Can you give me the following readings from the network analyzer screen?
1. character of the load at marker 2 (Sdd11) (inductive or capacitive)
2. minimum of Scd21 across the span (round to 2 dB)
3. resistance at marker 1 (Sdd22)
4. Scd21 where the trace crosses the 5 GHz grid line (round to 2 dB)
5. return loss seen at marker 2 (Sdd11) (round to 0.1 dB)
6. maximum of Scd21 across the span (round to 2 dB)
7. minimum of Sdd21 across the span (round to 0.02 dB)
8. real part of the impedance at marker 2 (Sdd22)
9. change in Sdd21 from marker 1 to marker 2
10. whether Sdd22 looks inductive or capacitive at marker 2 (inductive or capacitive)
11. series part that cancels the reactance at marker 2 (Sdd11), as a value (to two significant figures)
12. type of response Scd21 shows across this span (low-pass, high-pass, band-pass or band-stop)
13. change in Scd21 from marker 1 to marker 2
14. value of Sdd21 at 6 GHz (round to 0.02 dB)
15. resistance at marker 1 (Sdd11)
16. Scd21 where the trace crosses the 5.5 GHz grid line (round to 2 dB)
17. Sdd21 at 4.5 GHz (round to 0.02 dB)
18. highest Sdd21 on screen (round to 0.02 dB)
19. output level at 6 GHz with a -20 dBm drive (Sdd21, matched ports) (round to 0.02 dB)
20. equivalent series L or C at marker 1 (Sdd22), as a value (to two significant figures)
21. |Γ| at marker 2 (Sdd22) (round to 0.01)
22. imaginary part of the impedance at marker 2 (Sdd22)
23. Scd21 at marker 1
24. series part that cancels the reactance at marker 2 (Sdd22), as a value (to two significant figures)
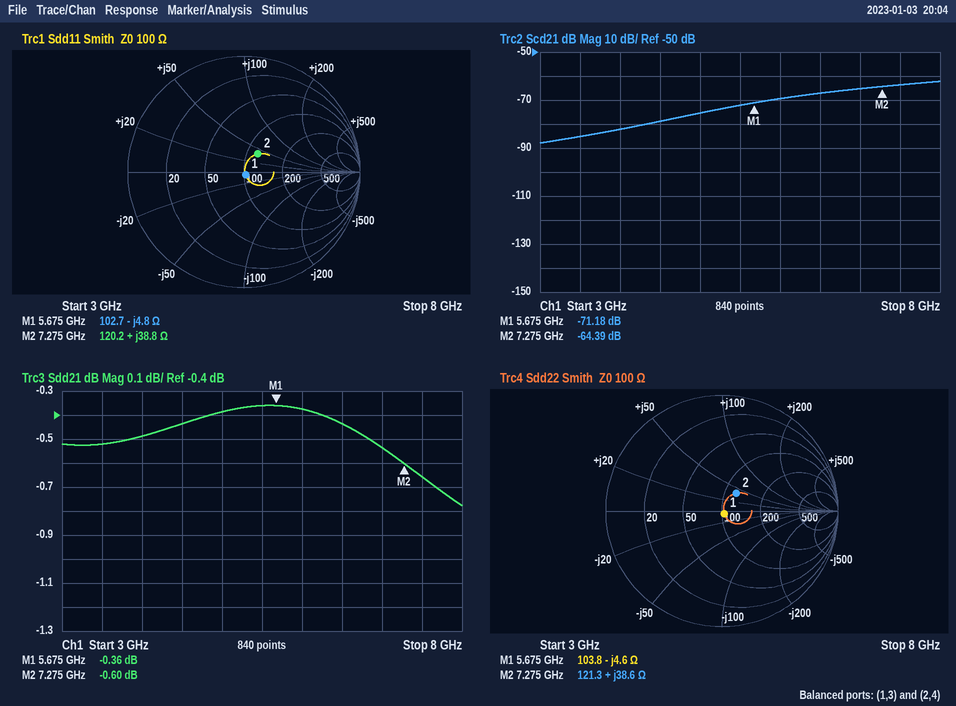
inductive
-88 dB
103.8 Ω
-76 dB
14.2 dB
-62 dB
-0.78 dB
121.3 Ω
-0.24 dB
inductive
560 fF
high-pass
6.79 dB
-0.38 dB
102.7 Ω
-72 dB
-0.44 dB
-0.36 dB
-20.38 dBm
6.1 pF
0.20
+38.6 Ω
-71.18 dB
570 fF
